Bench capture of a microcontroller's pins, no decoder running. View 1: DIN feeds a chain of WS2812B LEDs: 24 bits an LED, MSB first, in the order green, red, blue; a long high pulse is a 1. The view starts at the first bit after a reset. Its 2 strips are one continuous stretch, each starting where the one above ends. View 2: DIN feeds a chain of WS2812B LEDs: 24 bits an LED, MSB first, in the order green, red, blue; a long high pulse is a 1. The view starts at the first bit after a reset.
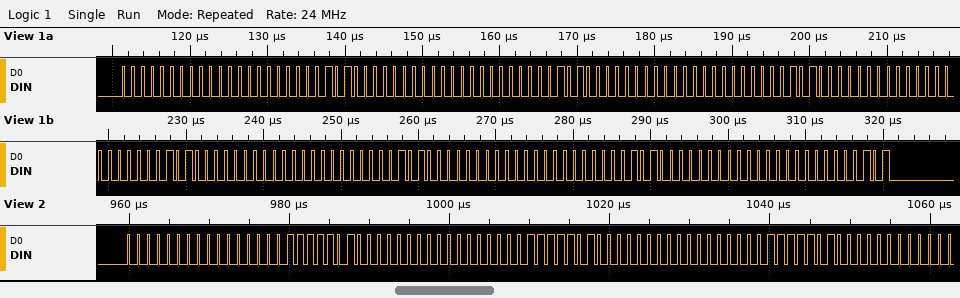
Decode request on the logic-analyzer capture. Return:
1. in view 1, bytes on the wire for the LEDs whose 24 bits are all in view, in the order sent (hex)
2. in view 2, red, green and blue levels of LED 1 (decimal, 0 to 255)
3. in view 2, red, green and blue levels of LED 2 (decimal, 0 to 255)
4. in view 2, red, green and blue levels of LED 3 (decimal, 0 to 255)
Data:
00 00 05 00 00 05 00 00 05 00 00 05 00 00 05 00 00 05 00 00 05
0, 0, 250
0, 0, 250
0, 0, 250
